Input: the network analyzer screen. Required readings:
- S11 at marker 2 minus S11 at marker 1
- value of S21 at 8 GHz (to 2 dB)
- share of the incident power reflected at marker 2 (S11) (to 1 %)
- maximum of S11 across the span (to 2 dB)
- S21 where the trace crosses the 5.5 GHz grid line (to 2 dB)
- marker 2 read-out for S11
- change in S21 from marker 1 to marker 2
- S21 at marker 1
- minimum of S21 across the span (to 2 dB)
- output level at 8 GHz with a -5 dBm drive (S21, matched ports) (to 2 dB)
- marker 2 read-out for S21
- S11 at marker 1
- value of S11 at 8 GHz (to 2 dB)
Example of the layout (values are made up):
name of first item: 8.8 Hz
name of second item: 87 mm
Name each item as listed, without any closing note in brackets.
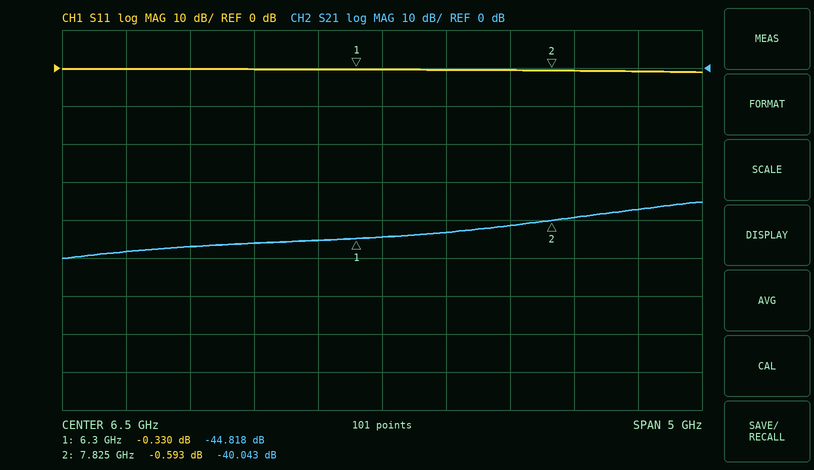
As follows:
S11 at marker 2 minus S11 at marker 1: -0.263 dB
value of S21 at 8 GHz: -40 dB
share of the incident power reflected at marker 2 (S11): 87 %
maximum of S11 across the span: 0 dB
S21 where the trace crosses the 5.5 GHz grid line: -46 dB
marker 2 read-out for S11: -0.593 dB
change in S21 from marker 1 to marker 2: 4.775 dB
S21 at marker 1: -44.818 dB
minimum of S21 across the span: -50 dB
output level at 8 GHz with a -5 dBm drive (S21, matched ports): -44 dBm
marker 2 read-out for S21: -40.043 dB
S11 at marker 1: -0.330 dB
value of S11 at 8 GHz: 0 dB
